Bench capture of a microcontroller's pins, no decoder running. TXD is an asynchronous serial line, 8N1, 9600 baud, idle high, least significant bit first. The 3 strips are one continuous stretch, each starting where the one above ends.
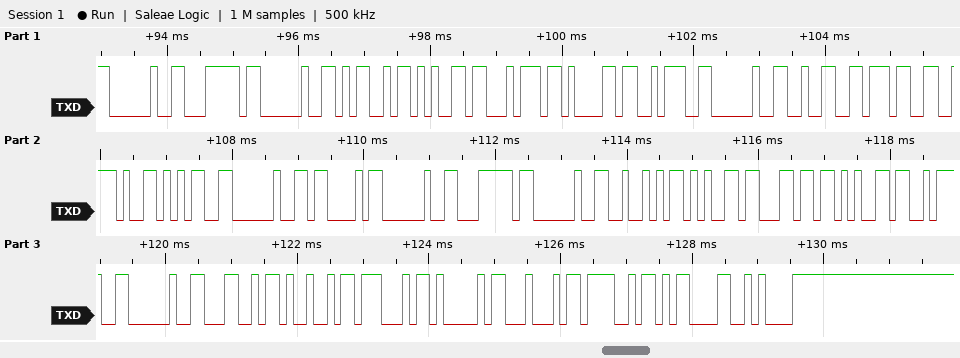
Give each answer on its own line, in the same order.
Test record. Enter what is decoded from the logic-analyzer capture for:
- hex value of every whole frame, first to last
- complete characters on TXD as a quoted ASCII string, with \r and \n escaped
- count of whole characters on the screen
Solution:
20 7C 20 4D 65 74 61 3A 20 32 37 2E 35 20 43 20 7C 20 52 65 6C 65 3A 20 4C 49 47 41 44 4F 0D 0A
" | Meta: 27.5 C | Rele: LIGADO\r\n"
32
